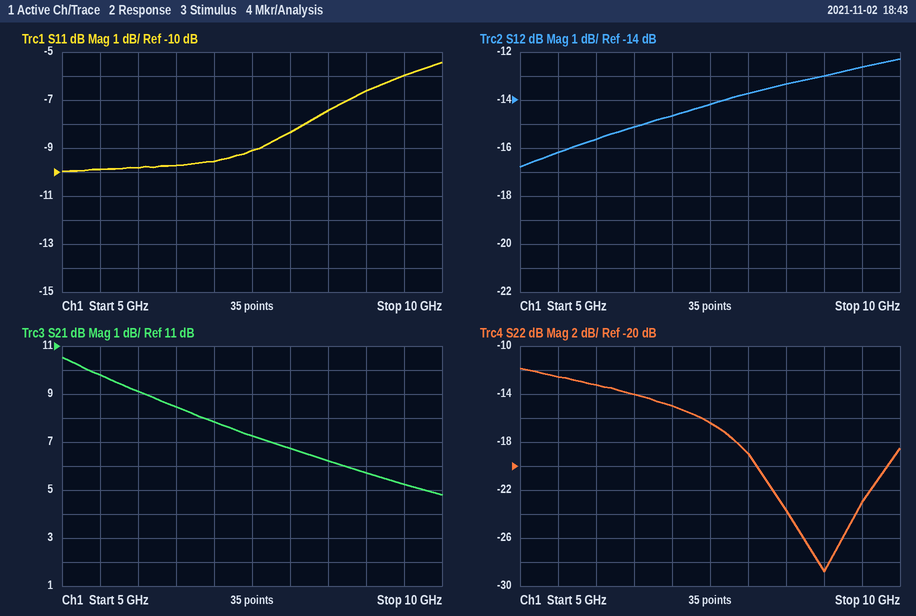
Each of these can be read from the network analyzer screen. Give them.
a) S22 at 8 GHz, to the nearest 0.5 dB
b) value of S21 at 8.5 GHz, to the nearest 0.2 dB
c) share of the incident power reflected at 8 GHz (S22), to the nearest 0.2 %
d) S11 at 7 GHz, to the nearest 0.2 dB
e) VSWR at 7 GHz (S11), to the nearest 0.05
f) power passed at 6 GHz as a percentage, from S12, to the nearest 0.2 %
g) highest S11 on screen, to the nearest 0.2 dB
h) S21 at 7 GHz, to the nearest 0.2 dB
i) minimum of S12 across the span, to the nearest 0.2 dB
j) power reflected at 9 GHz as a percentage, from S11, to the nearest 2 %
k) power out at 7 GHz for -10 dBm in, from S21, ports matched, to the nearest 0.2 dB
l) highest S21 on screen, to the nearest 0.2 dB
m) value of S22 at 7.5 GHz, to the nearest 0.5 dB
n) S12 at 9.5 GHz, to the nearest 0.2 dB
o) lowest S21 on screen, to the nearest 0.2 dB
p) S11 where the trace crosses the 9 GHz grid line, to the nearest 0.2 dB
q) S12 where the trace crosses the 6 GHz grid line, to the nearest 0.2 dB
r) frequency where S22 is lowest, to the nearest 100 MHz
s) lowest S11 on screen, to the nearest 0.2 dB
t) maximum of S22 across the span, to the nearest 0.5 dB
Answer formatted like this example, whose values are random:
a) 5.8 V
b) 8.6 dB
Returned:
a) -19.0 dB
b) 6.2 dB
c) 1.2 %
d) -9.6 dB
e) 2.00
f) 2.8 %
g) -5.4 dB
h) 7.8 dB
i) -16.8 dB
j) 22 %
k) -2.2 dBm
l) 10.6 dB
m) -16.5 dB
n) -12.6 dB
o) 4.8 dB
p) -6.6 dB
q) -15.6 dB
r) 9.0 GHz
s) -10.0 dB
t) -12.0 dB
